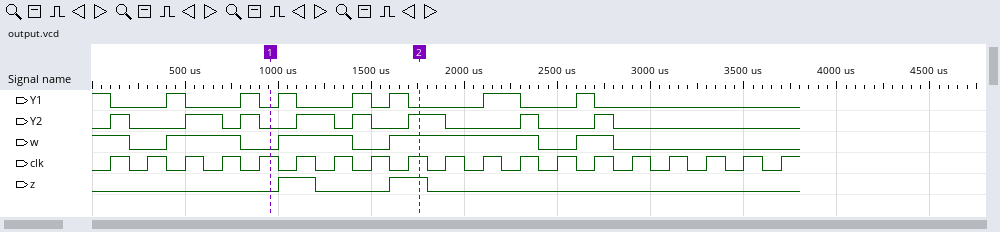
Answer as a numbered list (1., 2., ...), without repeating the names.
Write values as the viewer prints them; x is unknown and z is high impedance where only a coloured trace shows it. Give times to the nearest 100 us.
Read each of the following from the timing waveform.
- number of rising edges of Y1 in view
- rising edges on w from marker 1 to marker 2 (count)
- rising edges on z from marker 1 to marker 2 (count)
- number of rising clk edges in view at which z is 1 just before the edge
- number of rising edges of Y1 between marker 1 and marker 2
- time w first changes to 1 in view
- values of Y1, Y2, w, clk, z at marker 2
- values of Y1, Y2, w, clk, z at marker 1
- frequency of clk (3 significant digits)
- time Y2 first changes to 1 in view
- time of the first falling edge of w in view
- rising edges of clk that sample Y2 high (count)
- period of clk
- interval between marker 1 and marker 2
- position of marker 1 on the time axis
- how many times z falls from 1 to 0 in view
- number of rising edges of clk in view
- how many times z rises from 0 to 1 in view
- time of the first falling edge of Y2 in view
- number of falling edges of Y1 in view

1. 7
2. 2
3. 2
4. 2
5. 3
6. 400 us
7. Y1=0, Y2=1, w=1, clk=1, z=1
8. Y1=0, Y2=0, w=0, clk=1, z=0
9. 5.00 kHz
10. 100 us
11. 200 us
12. 5
13. 200 us
14. 800 us
15. 1000 us
16. 2
17. 19
18. 2
19. 200 us
20. 8
